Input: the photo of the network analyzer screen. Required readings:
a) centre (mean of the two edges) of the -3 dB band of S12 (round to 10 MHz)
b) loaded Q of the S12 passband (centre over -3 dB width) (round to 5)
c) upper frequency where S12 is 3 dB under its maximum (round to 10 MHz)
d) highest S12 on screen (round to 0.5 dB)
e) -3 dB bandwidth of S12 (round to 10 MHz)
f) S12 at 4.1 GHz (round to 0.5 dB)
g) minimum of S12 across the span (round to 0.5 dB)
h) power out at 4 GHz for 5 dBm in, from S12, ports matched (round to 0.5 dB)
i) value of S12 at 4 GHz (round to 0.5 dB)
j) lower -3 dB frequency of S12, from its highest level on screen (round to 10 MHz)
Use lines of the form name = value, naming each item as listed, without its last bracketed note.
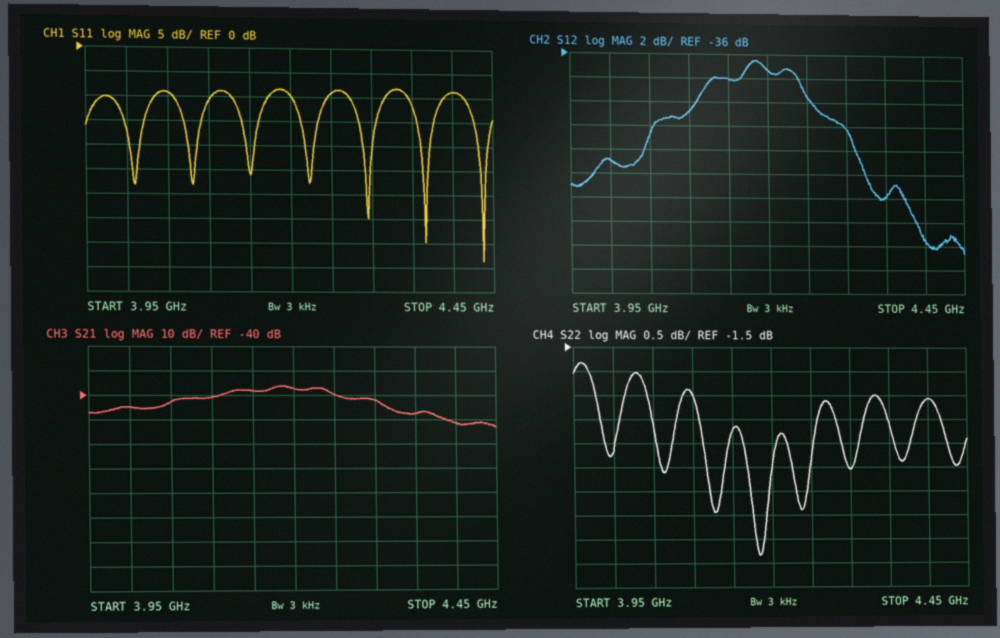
centre (mean of the two edges) of the -3 dB band of S12 = 4.18 GHz
loaded Q of the S12 passband (centre over -3 dB width) = 30
upper frequency where S12 is 3 dB under its maximum = 4.25 GHz
highest S12 on screen = -36.5 dB
-3 dB bandwidth of S12 = 140 MHz
S12 at 4.1 GHz = -41.0 dB
minimum of S12 across the span = -52.5 dB
power out at 4 GHz for 5 dBm in, from S12, ports matched = -40.0 dBm
value of S12 at 4 GHz = -45.0 dB
lower -3 dB frequency of S12, from its highest level on screen = 4.11 GHz
